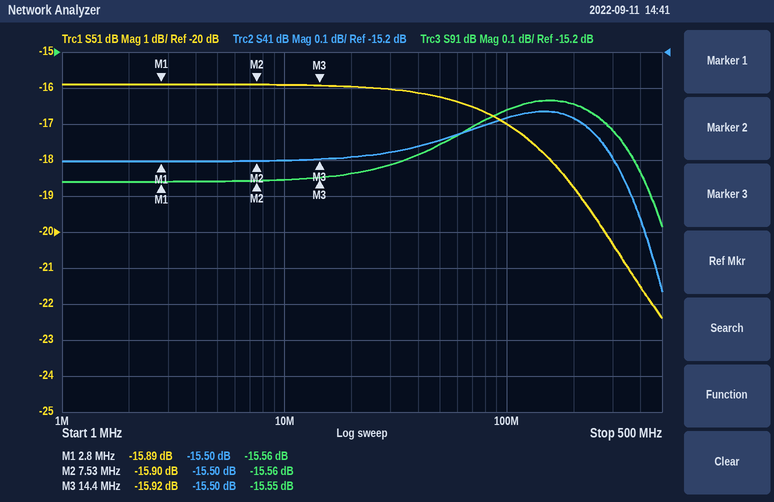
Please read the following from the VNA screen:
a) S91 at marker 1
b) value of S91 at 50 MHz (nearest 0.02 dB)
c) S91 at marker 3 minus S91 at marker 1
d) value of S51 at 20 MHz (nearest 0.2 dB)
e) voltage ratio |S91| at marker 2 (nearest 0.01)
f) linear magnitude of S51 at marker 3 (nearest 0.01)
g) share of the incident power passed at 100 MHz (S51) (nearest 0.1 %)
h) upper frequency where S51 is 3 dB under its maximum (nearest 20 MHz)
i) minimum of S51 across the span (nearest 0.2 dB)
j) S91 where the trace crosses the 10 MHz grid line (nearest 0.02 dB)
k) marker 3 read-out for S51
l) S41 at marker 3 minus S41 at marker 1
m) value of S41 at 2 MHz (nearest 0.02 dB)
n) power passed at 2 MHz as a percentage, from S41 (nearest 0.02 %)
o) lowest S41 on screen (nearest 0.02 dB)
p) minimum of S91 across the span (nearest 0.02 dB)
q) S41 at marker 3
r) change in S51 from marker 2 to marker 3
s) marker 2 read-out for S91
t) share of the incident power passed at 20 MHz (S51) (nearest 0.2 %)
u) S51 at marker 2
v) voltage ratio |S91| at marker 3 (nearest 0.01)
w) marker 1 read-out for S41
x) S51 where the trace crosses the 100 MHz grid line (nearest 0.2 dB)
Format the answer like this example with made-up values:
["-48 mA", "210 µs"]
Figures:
["-15.56 dB", "-15.46 dB", "0.01 dB", "-16.0 dB", "0.17", "0.16", "2.0 %", "200 MHz", "-22.4 dB", "-15.56 dB", "-15.92 dB", "0.00 dB", "-15.50 dB", "2.82 %", "-15.86 dB", "-15.68 dB", "-15.50 dB", "-0.02 dB", "-15.56 dB", "2.6 %", "-15.90 dB", "0.17", "-15.50 dB", "-17.0 dB"]
